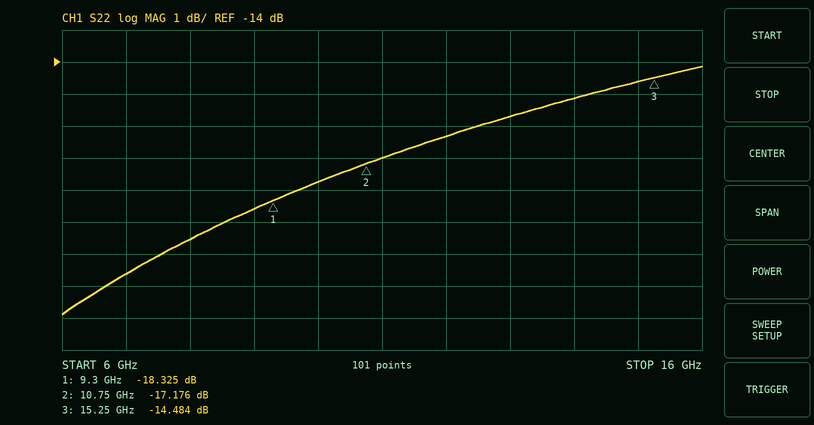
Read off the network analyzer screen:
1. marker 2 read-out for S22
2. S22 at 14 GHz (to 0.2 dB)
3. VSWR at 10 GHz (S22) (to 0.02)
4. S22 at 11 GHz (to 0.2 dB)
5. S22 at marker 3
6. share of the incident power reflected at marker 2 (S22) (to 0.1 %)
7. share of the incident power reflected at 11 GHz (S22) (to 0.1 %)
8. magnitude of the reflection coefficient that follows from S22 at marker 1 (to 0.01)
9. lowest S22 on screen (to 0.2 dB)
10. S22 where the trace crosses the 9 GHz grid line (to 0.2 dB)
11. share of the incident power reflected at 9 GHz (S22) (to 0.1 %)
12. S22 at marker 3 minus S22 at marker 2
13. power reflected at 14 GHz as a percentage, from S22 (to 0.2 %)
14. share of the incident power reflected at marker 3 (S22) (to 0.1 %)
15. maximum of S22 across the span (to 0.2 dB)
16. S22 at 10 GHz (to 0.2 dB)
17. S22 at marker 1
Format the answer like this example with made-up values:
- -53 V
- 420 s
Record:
- -17.176 dB
- -15.2 dB
- 1.30
- -17.0 dB
- -14.484 dB
- 1.9 %
- 2.0 %
- 0.12
- -21.8 dB
- -18.6 dB
- 1.4 %
- 2.692 dB
- 3.0 %
- 3.6 %
- -14.2 dB
- -17.8 dB
- -18.325 dB
